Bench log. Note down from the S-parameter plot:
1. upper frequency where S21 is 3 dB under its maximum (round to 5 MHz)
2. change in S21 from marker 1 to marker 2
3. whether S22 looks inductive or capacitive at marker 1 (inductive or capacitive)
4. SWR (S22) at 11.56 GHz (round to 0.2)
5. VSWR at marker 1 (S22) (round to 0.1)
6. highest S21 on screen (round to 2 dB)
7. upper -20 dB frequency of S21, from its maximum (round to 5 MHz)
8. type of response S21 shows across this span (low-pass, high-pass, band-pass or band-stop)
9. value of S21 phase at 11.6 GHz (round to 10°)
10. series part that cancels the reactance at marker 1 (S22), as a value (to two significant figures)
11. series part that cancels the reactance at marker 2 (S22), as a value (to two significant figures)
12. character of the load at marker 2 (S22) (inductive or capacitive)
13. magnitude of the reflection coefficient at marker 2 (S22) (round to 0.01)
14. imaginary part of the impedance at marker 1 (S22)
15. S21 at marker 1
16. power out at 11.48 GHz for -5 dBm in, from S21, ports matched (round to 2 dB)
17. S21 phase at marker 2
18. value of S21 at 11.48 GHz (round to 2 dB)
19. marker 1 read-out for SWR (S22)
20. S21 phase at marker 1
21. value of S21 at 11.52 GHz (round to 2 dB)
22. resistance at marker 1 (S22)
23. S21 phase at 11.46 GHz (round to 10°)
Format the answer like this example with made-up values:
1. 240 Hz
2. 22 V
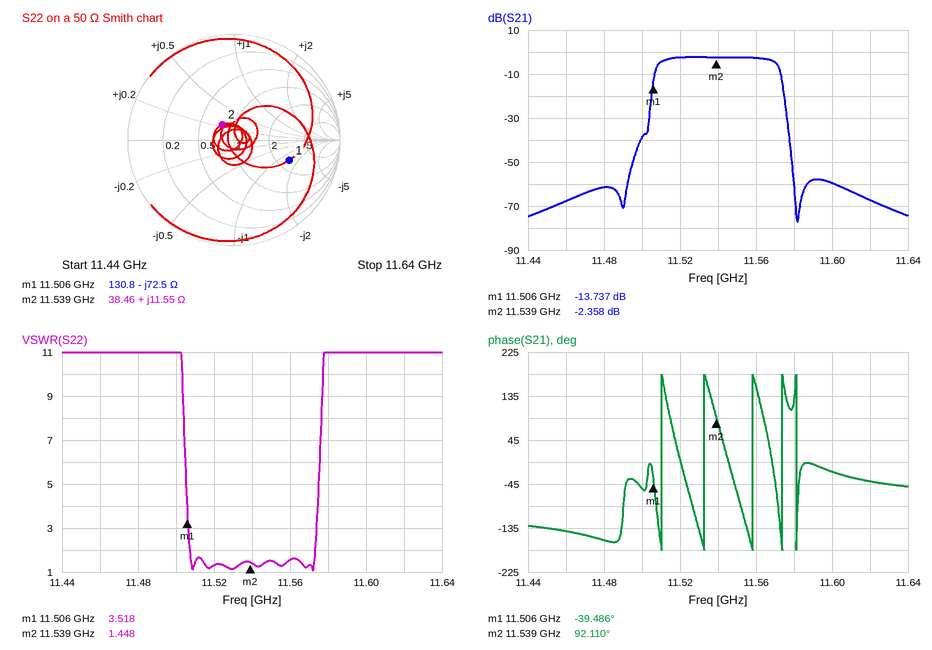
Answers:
1. 11.570 GHz
2. 11.379 dB
3. capacitive
4. 1.6
5. 3.5
6. -2 dB
7. 11.575 GHz
8. band-pass
9. -20°
10. 1.0 nH
11. 1.2 pF
12. inductive
13. 0.18
14. -72.5 Ω
15. -13.737 dB
16. -66 dBm
17. 92.110°
18. -62 dB
19. 3.518
20. -39.486°
21. -2 dB
22. 130.8 Ω
23. -140°
